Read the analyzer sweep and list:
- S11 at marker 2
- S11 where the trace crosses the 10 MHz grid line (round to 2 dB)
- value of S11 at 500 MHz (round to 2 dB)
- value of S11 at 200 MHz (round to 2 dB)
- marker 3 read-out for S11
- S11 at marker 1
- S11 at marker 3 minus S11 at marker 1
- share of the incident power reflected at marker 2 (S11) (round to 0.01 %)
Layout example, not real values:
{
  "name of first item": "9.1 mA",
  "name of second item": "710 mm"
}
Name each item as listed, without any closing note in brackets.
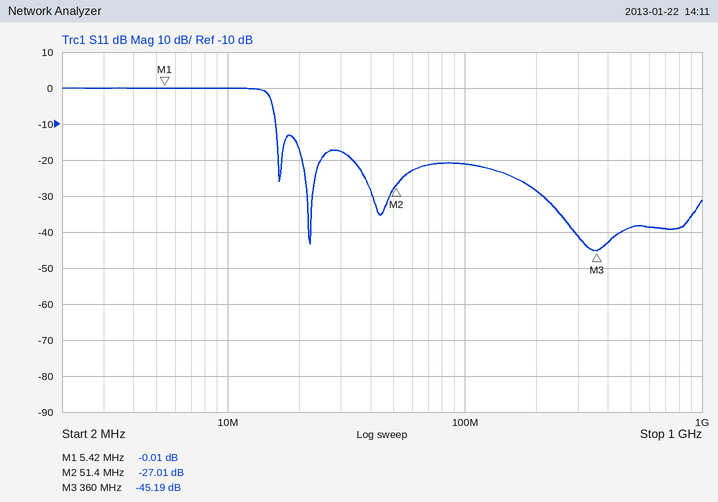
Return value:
{
  "S11 at marker 2": "-27.01 dB",
  "S11 where the trace crosses the 10 MHz grid line": "0 dB",
  "value of S11 at 500 MHz": "-38 dB",
  "value of S11 at 200 MHz": "-28 dB",
  "marker 3 read-out for S11": "-45.19 dB",
  "S11 at marker 1": "-0.01 dB",
  "S11 at marker 3 minus S11 at marker 1": "-45.18 dB",
  "share of the incident power reflected at marker 2 (S11)": "0.20 %"
}
